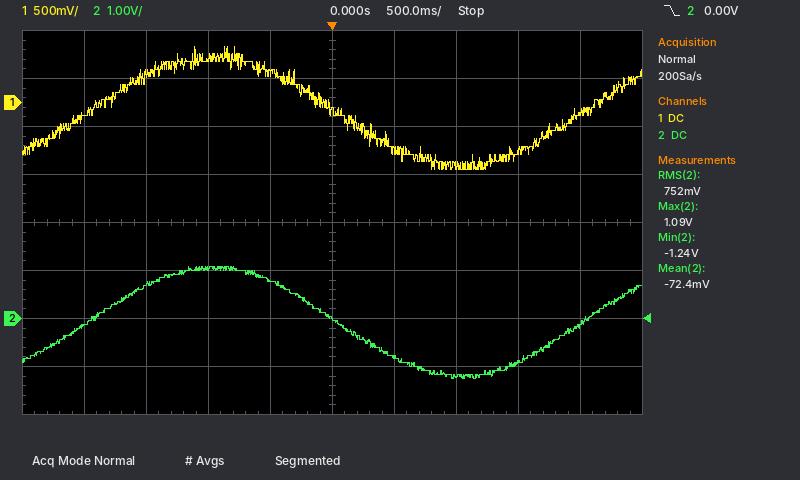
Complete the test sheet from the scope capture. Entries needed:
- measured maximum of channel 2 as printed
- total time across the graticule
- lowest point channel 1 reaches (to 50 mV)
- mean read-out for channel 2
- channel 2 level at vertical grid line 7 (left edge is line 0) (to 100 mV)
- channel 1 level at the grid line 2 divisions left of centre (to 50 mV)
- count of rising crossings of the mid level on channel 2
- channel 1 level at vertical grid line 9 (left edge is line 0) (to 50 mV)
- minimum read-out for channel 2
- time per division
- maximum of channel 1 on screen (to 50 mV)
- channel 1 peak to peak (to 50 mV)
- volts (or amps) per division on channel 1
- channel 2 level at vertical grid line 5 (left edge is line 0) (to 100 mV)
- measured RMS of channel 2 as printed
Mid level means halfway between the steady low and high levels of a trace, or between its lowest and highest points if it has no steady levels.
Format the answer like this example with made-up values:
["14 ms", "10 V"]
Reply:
["1.09 V", "5 s", "-700 mV", "-72.4 mV", "-1.2 V", "450 mV", "2", "-100 mV", "-1.24 V", "500 ms", "600 mV", "1.30 V", "500 mV", "0.0 V", "752 mV"]
